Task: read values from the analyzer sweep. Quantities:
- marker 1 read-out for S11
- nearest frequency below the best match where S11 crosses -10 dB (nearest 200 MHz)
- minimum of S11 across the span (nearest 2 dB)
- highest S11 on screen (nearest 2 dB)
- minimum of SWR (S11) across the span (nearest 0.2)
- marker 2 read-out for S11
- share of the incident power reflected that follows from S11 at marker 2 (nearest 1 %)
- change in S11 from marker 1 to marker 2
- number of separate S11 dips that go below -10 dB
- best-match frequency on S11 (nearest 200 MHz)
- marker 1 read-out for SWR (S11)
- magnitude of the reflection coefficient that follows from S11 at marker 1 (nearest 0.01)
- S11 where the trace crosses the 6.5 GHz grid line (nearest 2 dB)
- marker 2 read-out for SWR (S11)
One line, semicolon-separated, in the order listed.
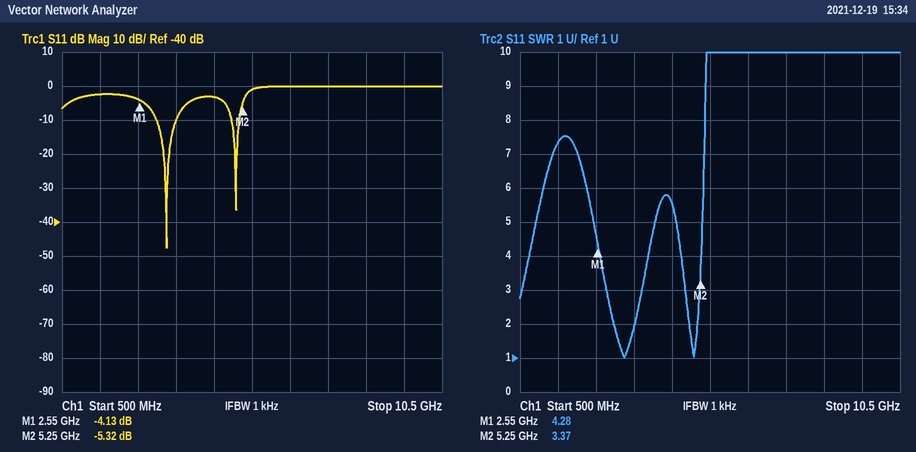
-4.13 dB; 3.0 GHz; -48 dB; 0 dB; 1.0; -5.32 dB; 29 %; -1.19 dB; 2; 3.2 GHz; 4.28; 0.62; 0 dB; 3.37
